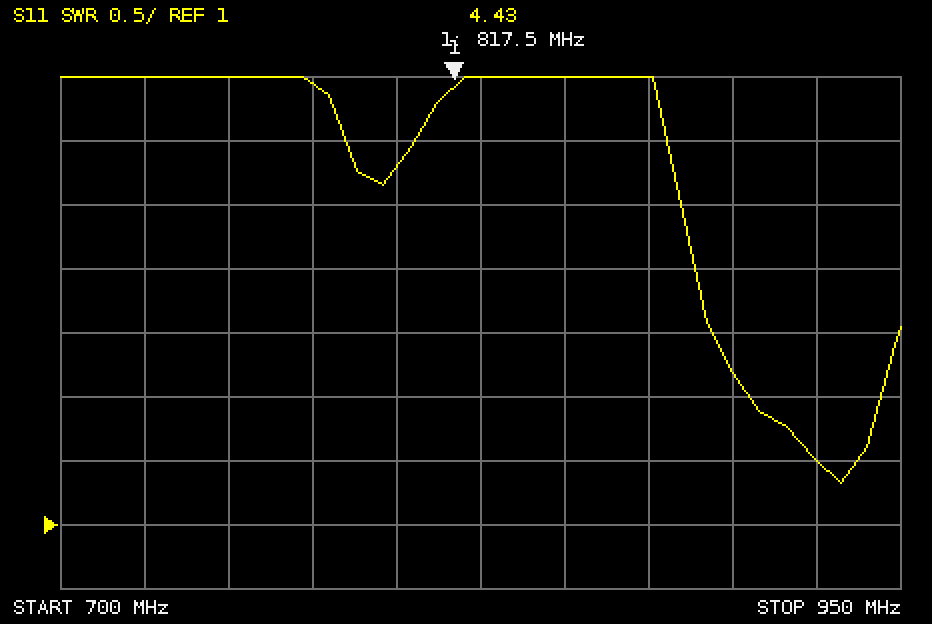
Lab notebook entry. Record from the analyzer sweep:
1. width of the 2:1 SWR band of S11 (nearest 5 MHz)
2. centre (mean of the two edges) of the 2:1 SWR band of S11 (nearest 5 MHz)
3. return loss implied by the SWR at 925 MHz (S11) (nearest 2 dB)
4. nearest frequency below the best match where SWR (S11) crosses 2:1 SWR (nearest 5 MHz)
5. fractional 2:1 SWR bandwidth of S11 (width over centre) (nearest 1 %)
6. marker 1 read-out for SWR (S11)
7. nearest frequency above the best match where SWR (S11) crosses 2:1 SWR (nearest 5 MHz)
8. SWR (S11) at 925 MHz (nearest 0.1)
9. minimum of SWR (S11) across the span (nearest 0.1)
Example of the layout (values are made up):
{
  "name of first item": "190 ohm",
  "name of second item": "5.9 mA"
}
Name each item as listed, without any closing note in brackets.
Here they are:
{
  "width of the 2:1 SWR band of S11": "40 MHz",
  "centre (mean of the two edges) of the 2:1 SWR band of S11": "925 MHz",
  "return loss implied by the SWR at 925 MHz (S11)": "14 dB",
  "nearest frequency below the best match where SWR (S11) crosses 2:1 SWR": "905 MHz",
  "fractional 2:1 SWR bandwidth of S11 (width over centre)": "4 %",
  "marker 1 read-out for SWR": "4.43",
  "nearest frequency above the best match where SWR (S11) crosses 2:1 SWR": "945 MHz",
  "SWR (S11) at 925 MHz": "1.5",
  "minimum of SWR (S11) across the span": "1.3"
}
